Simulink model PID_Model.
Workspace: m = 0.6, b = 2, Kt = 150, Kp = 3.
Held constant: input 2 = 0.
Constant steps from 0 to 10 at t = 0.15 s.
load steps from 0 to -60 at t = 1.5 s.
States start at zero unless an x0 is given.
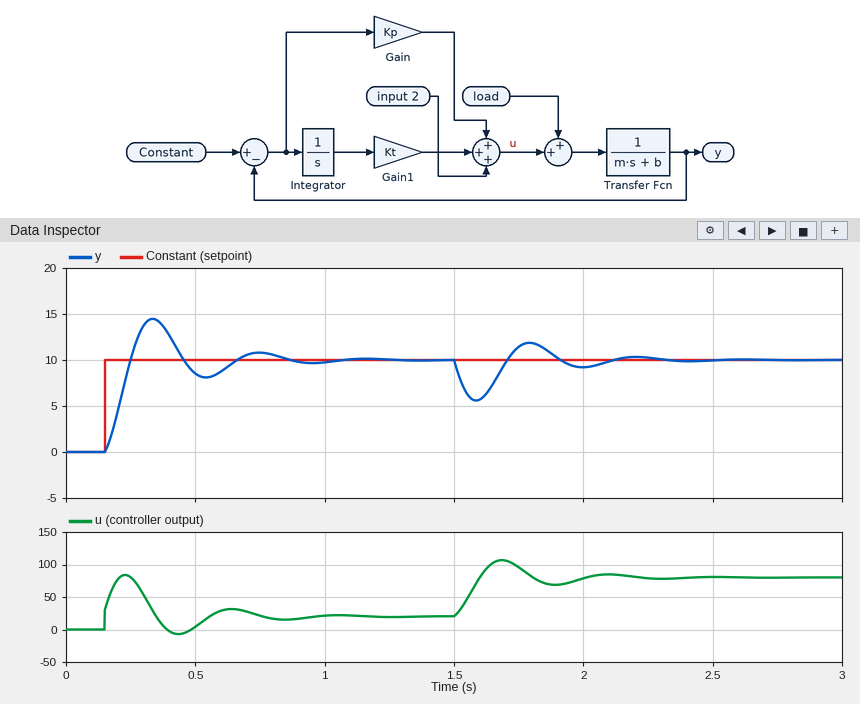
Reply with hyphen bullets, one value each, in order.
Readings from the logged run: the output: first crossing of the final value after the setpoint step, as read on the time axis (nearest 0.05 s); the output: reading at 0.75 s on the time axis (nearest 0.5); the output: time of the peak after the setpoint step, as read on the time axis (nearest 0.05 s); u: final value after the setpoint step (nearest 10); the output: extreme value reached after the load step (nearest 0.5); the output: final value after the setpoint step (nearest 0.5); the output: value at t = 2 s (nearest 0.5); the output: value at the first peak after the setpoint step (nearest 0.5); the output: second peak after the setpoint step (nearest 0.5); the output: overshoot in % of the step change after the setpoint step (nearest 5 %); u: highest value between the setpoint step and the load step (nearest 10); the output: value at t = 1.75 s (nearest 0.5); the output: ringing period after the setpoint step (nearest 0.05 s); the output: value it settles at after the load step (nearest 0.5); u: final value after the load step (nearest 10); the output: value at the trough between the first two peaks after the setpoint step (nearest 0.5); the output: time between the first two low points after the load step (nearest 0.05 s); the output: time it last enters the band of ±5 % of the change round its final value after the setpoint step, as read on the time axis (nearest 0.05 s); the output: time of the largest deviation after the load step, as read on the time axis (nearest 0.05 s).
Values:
- 0.25 s
- 11.0
- 0.35 s
- 20
- 5.5
- 10.0
- 9.0
- 14.5
- 11.0
- 45 %
- 80
- 11.5
- 0.40 s
- 10.0
- 80
- 8.0
- 0.40 s
- 0.80 s
- 1.60 s
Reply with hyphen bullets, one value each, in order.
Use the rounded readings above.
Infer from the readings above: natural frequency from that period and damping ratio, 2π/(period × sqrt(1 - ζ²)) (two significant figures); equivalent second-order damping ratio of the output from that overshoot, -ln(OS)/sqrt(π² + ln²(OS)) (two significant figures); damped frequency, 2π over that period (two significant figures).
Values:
- 16 rad/s
- 0.25
- 16 rad/s
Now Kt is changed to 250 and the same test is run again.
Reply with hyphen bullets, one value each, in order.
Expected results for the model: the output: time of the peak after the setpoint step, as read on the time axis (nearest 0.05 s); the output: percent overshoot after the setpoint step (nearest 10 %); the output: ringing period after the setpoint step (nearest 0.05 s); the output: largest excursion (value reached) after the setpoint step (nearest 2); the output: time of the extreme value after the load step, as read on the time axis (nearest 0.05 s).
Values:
- 0.30 s
- 50 %
- 0.30 s
- 16
- 1.55 s
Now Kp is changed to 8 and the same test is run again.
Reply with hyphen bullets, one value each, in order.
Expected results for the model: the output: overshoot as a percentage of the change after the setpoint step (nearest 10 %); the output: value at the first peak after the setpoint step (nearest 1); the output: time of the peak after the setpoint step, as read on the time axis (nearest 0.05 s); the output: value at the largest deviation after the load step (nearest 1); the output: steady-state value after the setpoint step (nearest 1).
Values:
- 20 %
- 12
- 0.30 s
- 7
- 10
